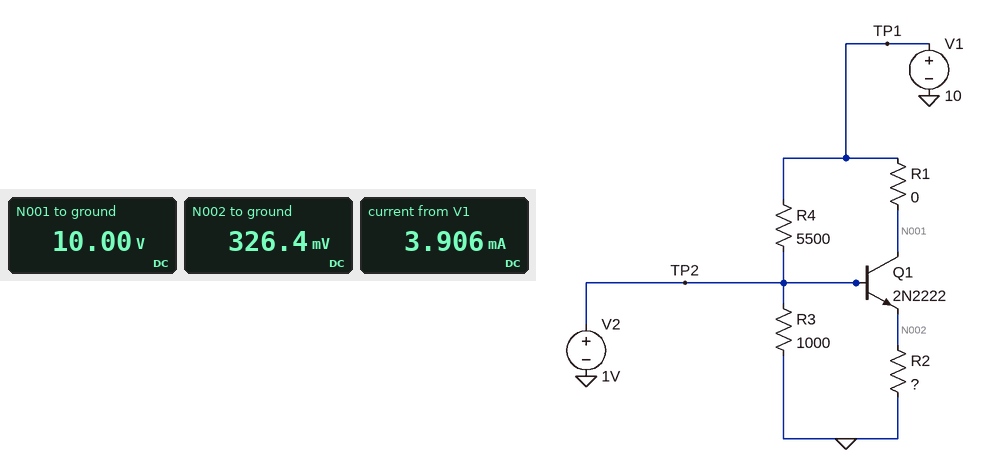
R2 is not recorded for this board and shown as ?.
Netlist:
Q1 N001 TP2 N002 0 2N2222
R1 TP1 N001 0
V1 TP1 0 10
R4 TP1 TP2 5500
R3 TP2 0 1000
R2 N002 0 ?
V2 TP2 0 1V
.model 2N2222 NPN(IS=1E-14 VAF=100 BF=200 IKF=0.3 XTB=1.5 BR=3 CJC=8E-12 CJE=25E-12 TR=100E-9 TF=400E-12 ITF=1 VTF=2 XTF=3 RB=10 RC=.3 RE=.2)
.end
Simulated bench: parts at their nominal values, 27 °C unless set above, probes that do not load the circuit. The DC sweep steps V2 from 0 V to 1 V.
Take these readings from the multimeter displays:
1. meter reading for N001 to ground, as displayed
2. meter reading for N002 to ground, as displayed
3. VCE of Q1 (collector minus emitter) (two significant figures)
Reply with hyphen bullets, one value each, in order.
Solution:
- 10.00 V
- 326.4 mV
- 9.7 V
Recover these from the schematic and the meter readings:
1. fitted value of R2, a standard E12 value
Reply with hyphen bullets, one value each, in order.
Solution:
- 150 Ω
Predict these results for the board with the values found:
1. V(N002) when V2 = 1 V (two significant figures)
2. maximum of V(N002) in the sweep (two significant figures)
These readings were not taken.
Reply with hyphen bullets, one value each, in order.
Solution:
- 330 mV
- 330 mV
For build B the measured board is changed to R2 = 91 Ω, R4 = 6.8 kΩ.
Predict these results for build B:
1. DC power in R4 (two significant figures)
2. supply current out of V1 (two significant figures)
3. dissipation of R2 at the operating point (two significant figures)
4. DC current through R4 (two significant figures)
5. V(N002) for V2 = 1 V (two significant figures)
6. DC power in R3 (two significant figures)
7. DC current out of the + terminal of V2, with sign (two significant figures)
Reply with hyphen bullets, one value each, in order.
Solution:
- 12 mW
- 5.9 mA
- 1.1 mW
- 1.3 mA
- 310 mV
- 1.0 mW
- -310 µA
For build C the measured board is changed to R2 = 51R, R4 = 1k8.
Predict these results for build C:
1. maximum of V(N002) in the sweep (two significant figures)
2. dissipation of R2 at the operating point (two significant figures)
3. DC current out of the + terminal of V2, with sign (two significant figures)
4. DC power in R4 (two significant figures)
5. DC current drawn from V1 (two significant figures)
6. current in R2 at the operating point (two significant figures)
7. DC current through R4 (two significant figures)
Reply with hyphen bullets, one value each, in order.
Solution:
- 300 mV
- 1.8 mW
- -4.0 mA
- 45 mW
- 12 mA
- 5.9 mA
- 5.0 mA
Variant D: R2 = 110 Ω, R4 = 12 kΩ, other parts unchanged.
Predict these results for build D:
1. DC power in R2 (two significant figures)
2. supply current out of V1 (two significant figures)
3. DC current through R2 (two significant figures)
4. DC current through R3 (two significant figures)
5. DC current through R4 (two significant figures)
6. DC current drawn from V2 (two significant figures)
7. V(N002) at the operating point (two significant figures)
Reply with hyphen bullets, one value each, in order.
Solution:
- 920 µW
- 5.9 mA
- 2.9 mA
- 1.0 mA
- 750 µA
- 260 µA
- 320 mV
